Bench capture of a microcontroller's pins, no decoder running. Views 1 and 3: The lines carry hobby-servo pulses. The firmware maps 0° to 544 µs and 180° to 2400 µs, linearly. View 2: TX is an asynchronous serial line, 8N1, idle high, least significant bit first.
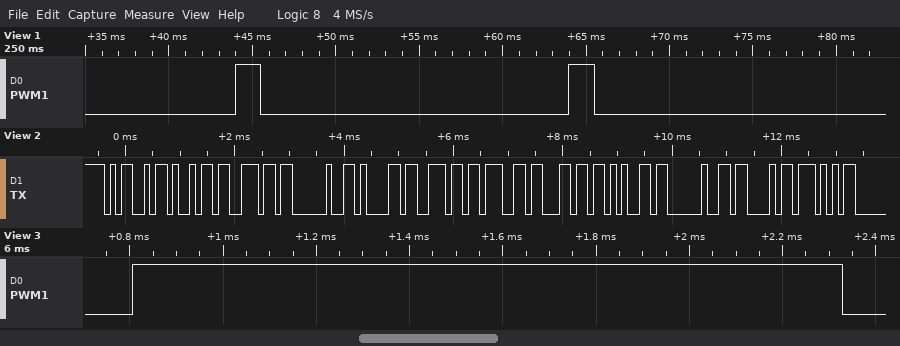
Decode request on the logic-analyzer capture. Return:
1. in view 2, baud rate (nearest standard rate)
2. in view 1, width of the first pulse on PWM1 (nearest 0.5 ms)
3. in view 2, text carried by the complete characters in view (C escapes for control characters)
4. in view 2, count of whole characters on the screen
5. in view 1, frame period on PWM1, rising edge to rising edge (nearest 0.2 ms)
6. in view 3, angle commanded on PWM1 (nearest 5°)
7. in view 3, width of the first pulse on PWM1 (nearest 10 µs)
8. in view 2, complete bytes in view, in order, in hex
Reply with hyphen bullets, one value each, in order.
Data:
- 9600 baud
- 1.5 ms
- "Min angle CW"
- 12
- 20.0 ms
- 95°
- 1520 µs
- 4D 69 6E 20 61 6E 67 6C 65 20 43 57
